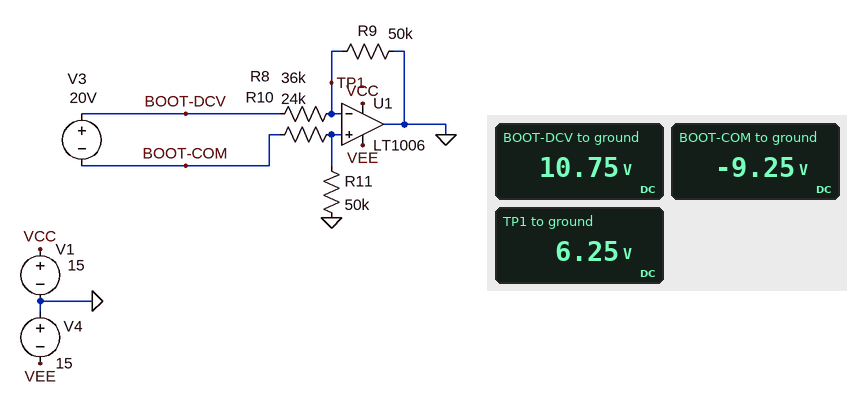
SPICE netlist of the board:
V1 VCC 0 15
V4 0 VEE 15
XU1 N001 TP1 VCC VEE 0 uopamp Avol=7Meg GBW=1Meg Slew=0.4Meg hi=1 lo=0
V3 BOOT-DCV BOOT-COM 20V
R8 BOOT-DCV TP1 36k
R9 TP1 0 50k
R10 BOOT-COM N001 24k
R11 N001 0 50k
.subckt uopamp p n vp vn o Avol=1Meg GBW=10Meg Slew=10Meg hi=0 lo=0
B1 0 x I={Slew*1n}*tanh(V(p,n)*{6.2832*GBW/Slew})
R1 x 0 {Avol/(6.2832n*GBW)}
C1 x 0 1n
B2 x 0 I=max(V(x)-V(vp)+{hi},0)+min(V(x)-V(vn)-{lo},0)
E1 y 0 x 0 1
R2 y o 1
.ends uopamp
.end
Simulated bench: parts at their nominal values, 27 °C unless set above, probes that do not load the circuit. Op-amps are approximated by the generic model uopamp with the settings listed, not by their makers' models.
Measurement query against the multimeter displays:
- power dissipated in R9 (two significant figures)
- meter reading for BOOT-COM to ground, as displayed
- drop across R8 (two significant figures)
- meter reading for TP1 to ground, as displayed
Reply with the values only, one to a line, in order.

780 µW
-9.25 V
4.5 V
6.25 V
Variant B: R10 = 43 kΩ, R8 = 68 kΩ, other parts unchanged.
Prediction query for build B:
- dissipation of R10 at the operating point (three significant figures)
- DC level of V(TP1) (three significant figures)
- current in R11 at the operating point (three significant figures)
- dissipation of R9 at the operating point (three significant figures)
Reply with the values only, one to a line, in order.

386 µW
4.74 V
94.8 µA
449 µW
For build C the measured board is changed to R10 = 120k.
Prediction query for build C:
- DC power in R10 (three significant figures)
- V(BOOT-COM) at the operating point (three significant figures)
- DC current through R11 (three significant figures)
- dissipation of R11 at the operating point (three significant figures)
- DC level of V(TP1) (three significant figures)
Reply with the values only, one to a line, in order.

732 µW
-13.3 V
78.1 µA
305 µW
3.91 V
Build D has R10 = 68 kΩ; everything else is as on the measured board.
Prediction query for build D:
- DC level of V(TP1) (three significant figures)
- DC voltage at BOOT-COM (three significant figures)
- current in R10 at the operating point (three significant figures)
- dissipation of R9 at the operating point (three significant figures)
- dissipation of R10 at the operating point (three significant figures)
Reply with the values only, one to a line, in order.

4.90 V
-11.6 V
98.0 µA
481 µW
654 µW
